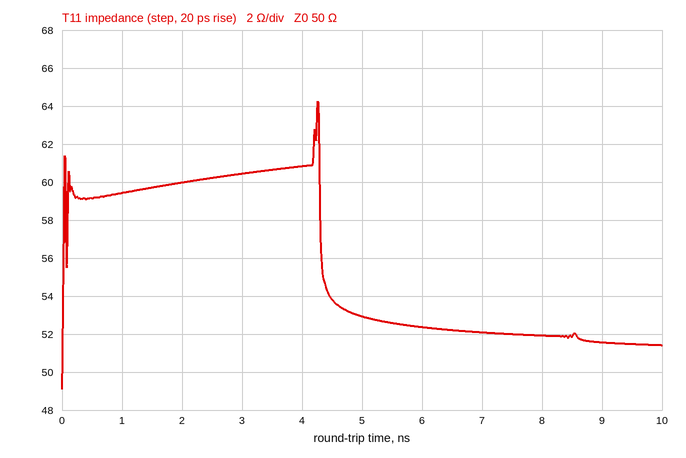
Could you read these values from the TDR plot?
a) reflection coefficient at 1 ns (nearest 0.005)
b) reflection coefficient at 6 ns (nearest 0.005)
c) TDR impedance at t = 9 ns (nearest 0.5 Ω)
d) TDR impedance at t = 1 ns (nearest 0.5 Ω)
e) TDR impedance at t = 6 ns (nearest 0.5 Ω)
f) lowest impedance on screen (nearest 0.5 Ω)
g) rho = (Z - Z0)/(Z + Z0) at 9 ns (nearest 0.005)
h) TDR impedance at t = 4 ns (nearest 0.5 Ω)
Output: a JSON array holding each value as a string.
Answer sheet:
["+0.085", "+0.025", "51.5 Ω", "59.5 Ω", "52.5 Ω", "49.0 Ω", "+0.015", "61.0 Ω"]
